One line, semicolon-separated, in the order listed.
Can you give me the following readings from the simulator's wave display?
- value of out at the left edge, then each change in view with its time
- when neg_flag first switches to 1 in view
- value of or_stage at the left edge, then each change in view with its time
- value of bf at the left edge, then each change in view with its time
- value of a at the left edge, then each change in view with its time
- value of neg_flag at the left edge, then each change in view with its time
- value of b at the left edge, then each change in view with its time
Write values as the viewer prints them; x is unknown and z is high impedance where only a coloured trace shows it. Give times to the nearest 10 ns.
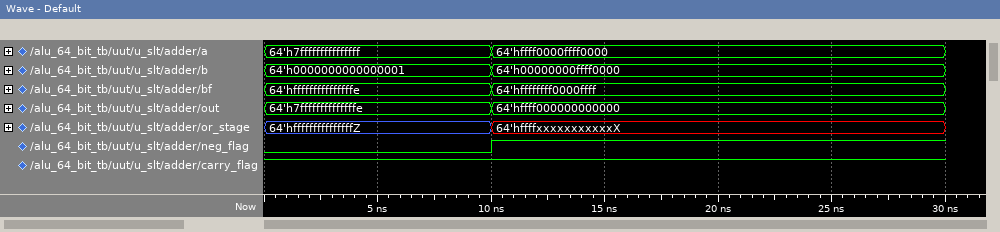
64'h7ffffffffffffffe, 64'hffff000000000000 at 10 ns; 10 ns; 64'hfffffffffffffffZ, 64'hffffxxxxxxxxxxxX at 10 ns; 64'hfffffffffffffffe, 64'hffffffff0000ffff at 10 ns; 64'h7fffffffffffffff, 64'hffff0000ffff0000 at 10 ns; 0, 1 at 10 ns; 64'h0000000000000001, 64'h00000000ffff0000 at 10 ns
